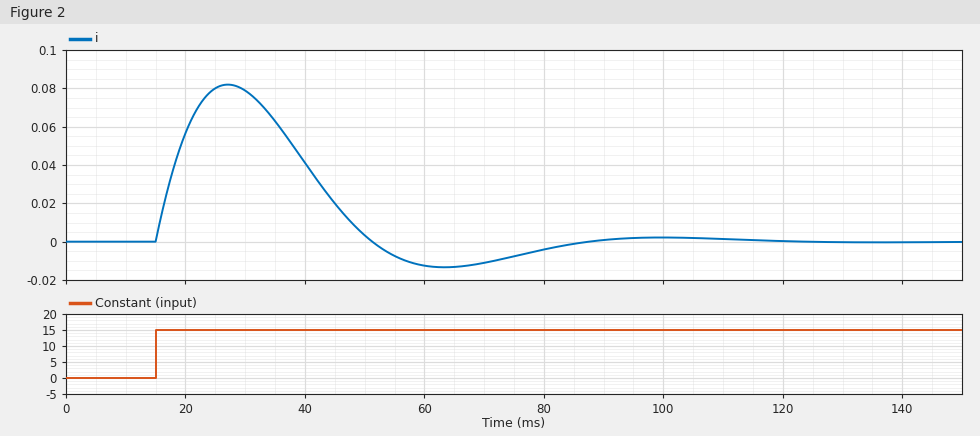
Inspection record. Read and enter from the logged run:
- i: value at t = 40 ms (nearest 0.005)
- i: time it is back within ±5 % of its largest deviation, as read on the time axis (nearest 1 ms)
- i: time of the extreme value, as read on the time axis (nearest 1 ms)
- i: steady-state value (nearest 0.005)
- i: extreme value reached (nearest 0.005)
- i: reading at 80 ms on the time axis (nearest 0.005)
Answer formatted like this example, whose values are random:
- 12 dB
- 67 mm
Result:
- 0.040
- 80 ms
- 27 ms
- 0.000
- 0.080
- -0.005
